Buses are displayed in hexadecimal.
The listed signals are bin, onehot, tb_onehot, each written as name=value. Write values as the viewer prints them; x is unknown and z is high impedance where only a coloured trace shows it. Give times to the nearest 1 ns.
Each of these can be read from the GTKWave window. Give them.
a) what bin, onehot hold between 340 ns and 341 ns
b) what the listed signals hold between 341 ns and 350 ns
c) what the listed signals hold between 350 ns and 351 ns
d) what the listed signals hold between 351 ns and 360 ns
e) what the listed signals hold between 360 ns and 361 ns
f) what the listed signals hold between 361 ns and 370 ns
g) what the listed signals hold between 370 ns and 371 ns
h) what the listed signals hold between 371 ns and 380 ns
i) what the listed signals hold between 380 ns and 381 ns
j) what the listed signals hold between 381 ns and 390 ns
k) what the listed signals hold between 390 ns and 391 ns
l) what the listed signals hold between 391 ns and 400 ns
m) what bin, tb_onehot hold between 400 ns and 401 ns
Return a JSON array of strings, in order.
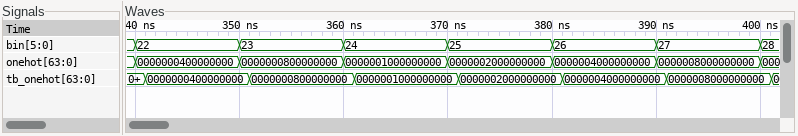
["bin=22, onehot=0000000400000000", "bin=22, onehot=0000000400000000, tb_onehot=0000000400000000", "bin=23, onehot=0000000800000000, tb_onehot=0000000400000000", "bin=23, onehot=0000000800000000, tb_onehot=0000000800000000", "bin=24, onehot=0000001000000000, tb_onehot=0000000800000000", "bin=24, onehot=0000001000000000, tb_onehot=0000001000000000", "bin=25, onehot=0000002000000000, tb_onehot=0000001000000000", "bin=25, onehot=0000002000000000, tb_onehot=0000002000000000", "bin=26, onehot=0000004000000000, tb_onehot=0000002000000000", "bin=26, onehot=0000004000000000, tb_onehot=0000004000000000", "bin=27, onehot=0000008000000000, tb_onehot=0000004000000000", "bin=27, onehot=0000008000000000, tb_onehot=0000008000000000", "bin=28, tb_onehot=0000008000000000"]
